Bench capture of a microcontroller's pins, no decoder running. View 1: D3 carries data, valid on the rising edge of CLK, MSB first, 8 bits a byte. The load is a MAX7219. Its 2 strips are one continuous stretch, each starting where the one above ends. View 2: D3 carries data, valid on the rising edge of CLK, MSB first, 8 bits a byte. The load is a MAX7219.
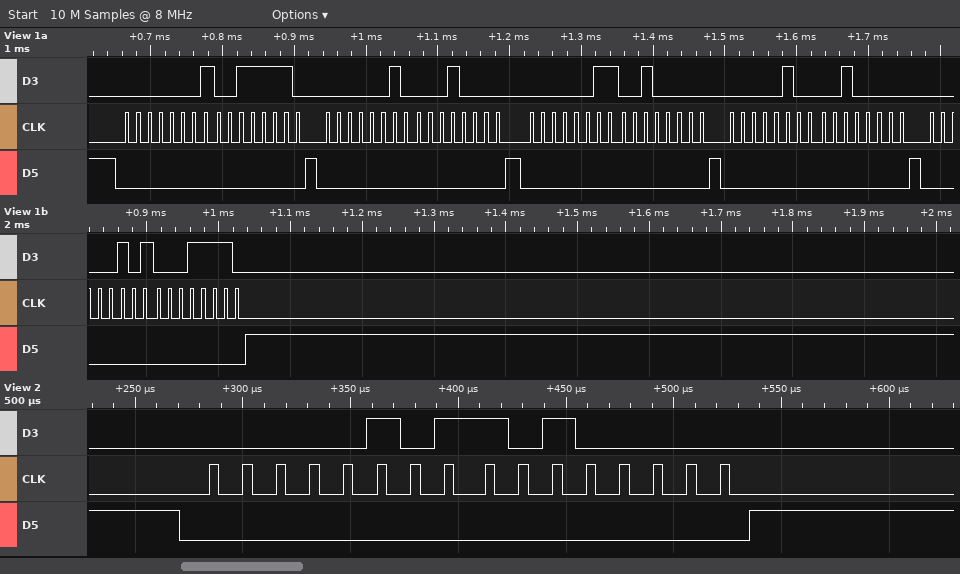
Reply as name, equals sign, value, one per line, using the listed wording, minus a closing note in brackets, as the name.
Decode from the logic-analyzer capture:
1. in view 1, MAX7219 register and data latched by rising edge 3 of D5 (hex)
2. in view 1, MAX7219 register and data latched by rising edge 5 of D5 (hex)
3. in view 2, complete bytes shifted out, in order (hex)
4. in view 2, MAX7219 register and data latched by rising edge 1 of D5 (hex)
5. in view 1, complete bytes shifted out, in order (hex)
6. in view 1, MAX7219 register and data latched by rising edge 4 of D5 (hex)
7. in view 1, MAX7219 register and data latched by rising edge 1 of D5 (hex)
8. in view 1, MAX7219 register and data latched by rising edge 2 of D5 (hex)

in view 1, MAX7219 register and data latched by rising edge 3 of D5 = register 0x3, data 0x20
in view 1, MAX7219 register and data latched by rising edge 5 of D5 = register 0x5, data 0x1E
in view 2, complete bytes shifted out, in order = 05 A0
in view 2, MAX7219 register and data latched by rising edge 1 of D5 = register 0x5, data 0xA0
in view 1, complete bytes shifted out, in order = 0x01 0x3E 0x02 0x10 0x03 0x20 0x04 0x20 0x05 0x1E
in view 1, MAX7219 register and data latched by rising edge 4 of D5 = register 0x4, data 0x20
in view 1, MAX7219 register and data latched by rising edge 1 of D5 = register 0x1, data 0x3E
in view 1, MAX7219 register and data latched by rising edge 2 of D5 = register 0x2, data 0x10
